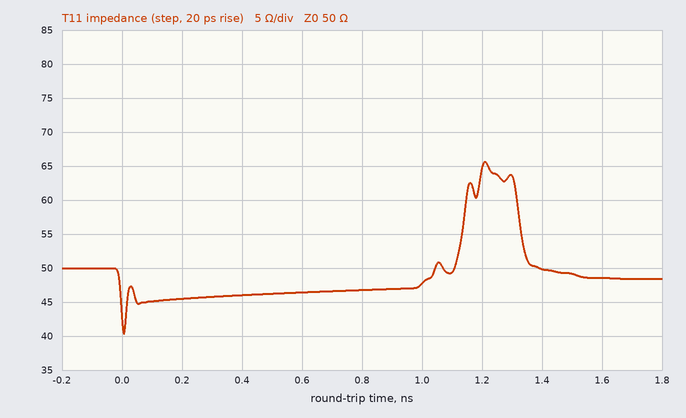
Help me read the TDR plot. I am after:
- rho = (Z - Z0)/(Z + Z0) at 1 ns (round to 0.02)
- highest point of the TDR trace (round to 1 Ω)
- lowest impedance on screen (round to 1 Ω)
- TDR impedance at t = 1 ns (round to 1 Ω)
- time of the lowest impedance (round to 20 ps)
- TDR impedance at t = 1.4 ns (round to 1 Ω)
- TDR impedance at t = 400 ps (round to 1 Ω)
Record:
-0.02
66 Ω
40 Ω
48 Ω
0 ps
50 Ω
46 Ω
